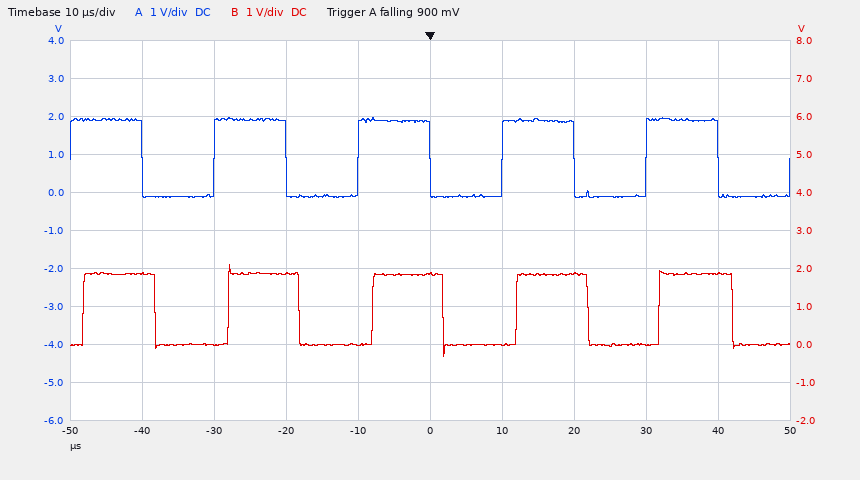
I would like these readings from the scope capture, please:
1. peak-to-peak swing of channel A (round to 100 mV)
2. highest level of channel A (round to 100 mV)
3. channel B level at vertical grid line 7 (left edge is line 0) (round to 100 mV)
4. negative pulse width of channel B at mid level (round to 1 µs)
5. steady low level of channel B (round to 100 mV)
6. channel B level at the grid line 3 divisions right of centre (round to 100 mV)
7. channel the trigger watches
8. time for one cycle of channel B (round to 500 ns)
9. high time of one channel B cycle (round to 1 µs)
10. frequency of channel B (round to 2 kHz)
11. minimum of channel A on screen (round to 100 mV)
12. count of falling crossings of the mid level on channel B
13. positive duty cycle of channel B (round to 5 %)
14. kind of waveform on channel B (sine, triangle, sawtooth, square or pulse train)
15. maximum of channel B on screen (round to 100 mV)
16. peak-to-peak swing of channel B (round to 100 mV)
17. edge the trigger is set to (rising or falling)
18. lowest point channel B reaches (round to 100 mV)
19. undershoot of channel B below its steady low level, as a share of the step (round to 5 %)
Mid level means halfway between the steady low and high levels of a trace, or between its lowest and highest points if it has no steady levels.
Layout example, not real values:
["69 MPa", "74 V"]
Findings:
["2.1 V", "2.0 V", "1.9 V", "10 µs", "0.0 V", "0.0 V", "channel A", "20.0 µs", "10 µs", "50 kHz", "-100 mV", "5", "50 %", "square", "2.1 V", "2.4 V", "falling", "-300 mV", "15 %"]
